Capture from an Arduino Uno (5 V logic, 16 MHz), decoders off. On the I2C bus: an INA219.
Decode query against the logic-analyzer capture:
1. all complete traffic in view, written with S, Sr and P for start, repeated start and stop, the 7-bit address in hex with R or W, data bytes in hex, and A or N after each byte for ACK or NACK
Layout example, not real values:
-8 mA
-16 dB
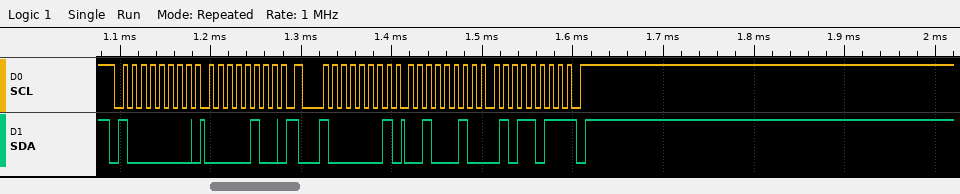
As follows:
S 40W A 04 A Sr 40R A 22 A 5B N P
